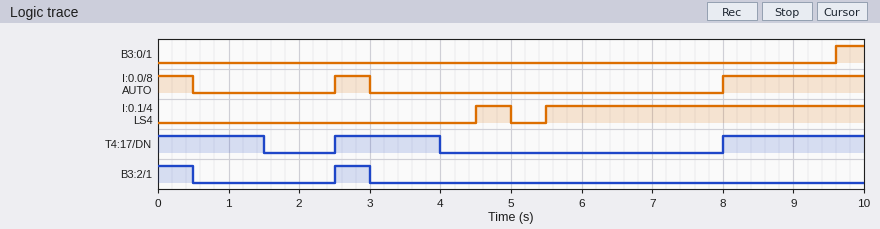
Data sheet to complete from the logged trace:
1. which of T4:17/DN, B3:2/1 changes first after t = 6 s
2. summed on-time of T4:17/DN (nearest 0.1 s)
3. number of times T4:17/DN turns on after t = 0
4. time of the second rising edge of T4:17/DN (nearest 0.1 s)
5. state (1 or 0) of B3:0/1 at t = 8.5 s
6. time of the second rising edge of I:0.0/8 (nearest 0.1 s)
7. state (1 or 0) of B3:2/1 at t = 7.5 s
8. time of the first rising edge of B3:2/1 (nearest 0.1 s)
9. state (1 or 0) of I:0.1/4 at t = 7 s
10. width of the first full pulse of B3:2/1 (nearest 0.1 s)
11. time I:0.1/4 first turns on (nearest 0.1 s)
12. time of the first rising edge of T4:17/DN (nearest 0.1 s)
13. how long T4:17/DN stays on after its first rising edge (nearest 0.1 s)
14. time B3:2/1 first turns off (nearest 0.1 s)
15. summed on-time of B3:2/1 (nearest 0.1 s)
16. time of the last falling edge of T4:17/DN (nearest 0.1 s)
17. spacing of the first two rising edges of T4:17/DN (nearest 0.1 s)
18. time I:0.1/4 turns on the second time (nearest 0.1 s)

T4:17/DN
5.0 s
2
8.0 s
0
8.0 s
0
2.5 s
1
0.5 s
4.5 s
2.5 s
1.5 s
0.5 s
1.0 s
4.0 s
5.5 s
5.5 s
